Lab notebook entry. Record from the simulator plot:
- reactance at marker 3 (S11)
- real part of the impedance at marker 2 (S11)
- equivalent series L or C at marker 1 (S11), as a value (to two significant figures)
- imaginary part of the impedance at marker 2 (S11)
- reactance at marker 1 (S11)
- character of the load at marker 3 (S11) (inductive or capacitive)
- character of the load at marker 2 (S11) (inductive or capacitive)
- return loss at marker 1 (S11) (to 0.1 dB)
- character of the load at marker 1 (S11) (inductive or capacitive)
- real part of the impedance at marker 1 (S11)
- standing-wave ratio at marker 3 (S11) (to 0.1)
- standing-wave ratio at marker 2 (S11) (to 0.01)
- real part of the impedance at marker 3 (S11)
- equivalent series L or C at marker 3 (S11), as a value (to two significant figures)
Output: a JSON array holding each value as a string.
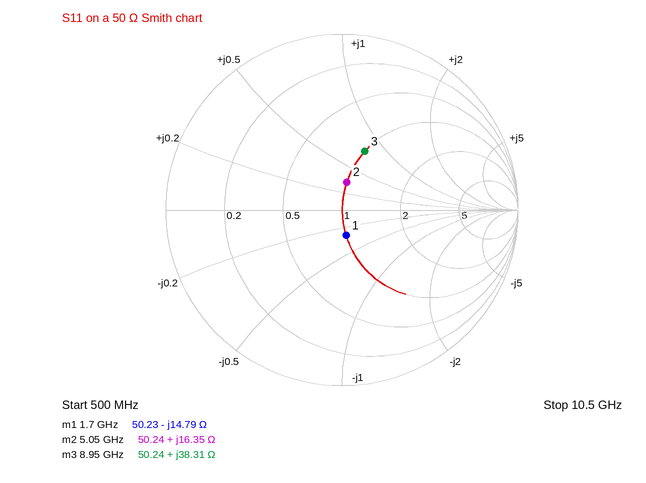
["+38.31 Ω", "50.24 Ω", "6.3 pF", "+16.35 Ω", "-14.79 Ω", "inductive", "inductive", "16.7 dB", "capacitive", "50.23 Ω", "2.1", "1.38", "50.24 Ω", "680 pH"]
